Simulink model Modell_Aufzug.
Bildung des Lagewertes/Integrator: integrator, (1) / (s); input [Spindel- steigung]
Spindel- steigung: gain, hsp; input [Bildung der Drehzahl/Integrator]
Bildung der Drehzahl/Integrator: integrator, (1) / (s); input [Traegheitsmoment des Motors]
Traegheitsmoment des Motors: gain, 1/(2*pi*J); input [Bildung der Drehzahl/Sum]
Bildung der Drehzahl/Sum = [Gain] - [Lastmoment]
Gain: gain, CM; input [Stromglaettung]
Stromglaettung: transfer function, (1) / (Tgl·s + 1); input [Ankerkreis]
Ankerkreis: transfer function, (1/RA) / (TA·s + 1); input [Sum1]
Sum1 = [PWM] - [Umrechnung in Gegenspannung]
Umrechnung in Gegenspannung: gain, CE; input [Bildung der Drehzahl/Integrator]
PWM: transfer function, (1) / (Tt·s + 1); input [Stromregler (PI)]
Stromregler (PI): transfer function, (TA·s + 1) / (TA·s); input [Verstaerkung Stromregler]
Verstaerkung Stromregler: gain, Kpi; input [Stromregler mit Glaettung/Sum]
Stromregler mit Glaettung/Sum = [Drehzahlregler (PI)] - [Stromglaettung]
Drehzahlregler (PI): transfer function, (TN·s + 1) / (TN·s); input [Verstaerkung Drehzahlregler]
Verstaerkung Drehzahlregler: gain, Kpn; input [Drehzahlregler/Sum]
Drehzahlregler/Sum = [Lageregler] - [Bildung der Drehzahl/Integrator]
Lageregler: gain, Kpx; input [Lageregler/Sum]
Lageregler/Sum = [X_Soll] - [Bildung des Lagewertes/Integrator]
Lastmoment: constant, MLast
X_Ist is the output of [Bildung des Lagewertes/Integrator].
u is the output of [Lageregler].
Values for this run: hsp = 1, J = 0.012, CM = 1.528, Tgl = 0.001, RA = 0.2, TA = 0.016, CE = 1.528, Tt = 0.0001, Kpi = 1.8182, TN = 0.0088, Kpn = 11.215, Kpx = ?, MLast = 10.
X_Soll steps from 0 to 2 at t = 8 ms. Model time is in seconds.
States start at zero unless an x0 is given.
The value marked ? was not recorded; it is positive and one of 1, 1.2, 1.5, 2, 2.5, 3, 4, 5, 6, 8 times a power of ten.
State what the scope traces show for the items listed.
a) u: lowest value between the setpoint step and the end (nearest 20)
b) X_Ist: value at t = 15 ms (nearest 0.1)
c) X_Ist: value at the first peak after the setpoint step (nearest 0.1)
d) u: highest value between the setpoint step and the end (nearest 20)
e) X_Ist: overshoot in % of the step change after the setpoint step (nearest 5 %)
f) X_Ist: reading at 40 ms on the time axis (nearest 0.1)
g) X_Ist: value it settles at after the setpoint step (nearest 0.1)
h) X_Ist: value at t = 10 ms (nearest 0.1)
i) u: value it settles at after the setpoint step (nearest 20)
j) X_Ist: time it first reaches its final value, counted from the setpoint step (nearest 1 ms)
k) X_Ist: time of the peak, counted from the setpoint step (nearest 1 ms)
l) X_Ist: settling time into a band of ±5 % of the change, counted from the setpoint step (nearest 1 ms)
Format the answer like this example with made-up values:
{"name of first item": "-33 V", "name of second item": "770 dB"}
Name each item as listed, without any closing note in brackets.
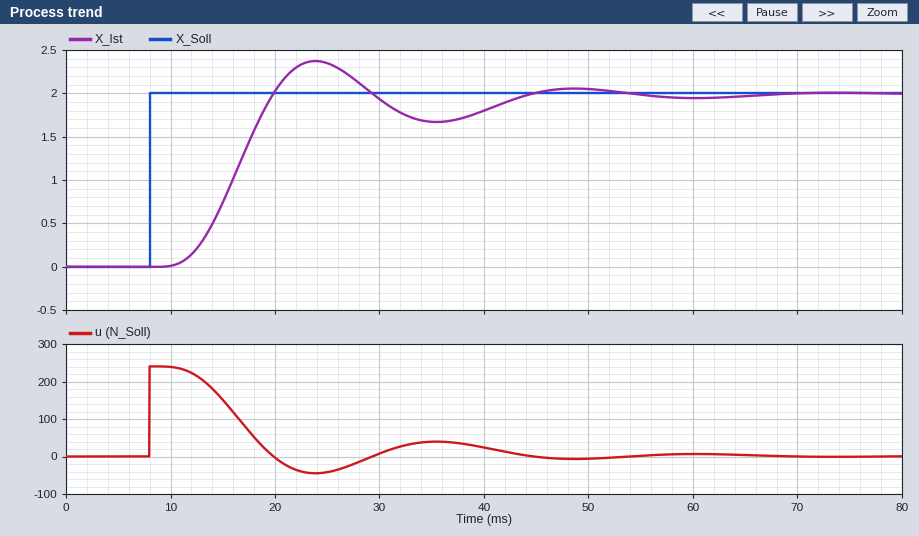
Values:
{"u: lowest value between the setpoint step and the end": "-40", "X_Ist: value at t = 15 ms": "0.7", "X_Ist: value at the first peak after the setpoint step": "2.4", "u: highest value between the setpoint step and the end": "240", "X_Ist: overshoot in % of the step change after the setpoint step": "20 %", "X_Ist: reading at 40 ms on the time axis": "1.8", "X_Ist: value it settles at after the setpoint step": "2.0", "X_Ist: value at t = 10 ms": "0.0", "u: value it settles at after the setpoint step": "0", "X_Ist: time it first reaches its final value, counted from the setpoint step": "12 ms", "X_Ist: time of the peak, counted from the setpoint step": "16 ms", "X_Ist: settling time into a band of ±5 % of the change, counted from the setpoint step": "34 ms"}
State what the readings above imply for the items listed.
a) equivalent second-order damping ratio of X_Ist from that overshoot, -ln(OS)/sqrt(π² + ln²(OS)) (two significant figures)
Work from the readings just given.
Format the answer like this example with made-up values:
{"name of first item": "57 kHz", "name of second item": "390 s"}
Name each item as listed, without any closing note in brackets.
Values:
{"equivalent second-order damping ratio of X_Ist from that overshoot, -ln(OS)/sqrt(π² + ln²(OS))": "0.46"}
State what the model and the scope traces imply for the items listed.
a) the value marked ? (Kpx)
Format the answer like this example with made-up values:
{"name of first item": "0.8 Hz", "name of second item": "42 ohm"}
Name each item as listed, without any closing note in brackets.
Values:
{"the value marked ?": "120"}
